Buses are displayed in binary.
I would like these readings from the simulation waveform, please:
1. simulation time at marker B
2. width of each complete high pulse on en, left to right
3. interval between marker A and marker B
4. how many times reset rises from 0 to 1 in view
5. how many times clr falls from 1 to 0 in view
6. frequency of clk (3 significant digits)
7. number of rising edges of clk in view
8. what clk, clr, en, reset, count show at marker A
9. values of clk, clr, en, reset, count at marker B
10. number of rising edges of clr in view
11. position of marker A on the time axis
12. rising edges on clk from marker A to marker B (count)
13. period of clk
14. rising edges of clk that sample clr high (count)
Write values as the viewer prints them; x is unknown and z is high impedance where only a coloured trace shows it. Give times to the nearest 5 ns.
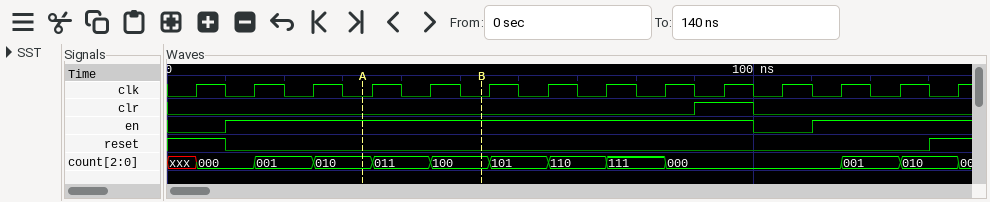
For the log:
55 ns
90 ns
20 ns
1
1
100 MHz
14
clk=0, clr=0, en=1, reset=0, count=010
clk=0, clr=0, en=1, reset=0, count=100
1
35 ns
2
10 ns
1
